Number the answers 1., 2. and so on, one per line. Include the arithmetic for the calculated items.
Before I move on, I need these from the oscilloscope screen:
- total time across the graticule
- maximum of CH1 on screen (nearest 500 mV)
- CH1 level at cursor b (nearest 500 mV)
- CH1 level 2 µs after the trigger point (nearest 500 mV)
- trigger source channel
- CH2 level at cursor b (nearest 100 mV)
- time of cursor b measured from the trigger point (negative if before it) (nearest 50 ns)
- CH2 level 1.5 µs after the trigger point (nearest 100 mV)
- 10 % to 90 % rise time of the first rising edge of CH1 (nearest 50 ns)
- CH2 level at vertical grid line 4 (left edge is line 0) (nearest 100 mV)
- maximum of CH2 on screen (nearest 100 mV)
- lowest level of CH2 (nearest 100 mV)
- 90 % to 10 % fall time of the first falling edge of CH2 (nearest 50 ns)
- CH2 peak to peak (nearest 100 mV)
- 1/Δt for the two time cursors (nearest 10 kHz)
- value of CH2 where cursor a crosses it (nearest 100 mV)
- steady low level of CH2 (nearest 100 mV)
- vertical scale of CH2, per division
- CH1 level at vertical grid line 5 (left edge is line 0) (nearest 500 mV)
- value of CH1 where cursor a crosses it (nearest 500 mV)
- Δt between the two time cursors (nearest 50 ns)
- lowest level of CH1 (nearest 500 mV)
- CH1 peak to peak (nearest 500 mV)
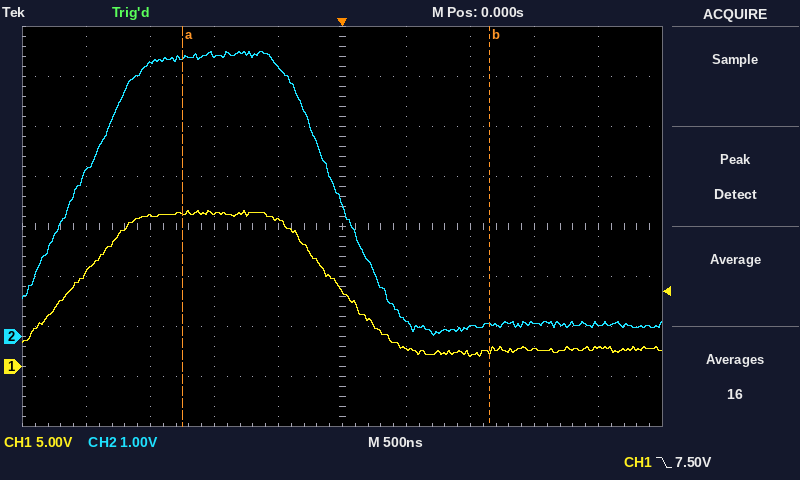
1. 5 µs
2. 15.5 V
3. 1.5 V
4. 2.0 V
5. CH1
6. 200 mV
7. +1.15 µs
8. 300 mV
9. 750 ns
10. 5.4 V
11. 5.7 V
12. 0.0 V
13. 750 ns
14. 5.7 V − (0.0 V) = 5.7 V
15. 1 / 2.40 µs ≈ 420 kHz
16. 5.6 V
17. 200 mV
18. 1 V
19. 7.5 V
20. 15.5 V
21. 2.40 µs
22. 1.0 V
23. 15.5 V − (1.0 V) = 14.5 V
